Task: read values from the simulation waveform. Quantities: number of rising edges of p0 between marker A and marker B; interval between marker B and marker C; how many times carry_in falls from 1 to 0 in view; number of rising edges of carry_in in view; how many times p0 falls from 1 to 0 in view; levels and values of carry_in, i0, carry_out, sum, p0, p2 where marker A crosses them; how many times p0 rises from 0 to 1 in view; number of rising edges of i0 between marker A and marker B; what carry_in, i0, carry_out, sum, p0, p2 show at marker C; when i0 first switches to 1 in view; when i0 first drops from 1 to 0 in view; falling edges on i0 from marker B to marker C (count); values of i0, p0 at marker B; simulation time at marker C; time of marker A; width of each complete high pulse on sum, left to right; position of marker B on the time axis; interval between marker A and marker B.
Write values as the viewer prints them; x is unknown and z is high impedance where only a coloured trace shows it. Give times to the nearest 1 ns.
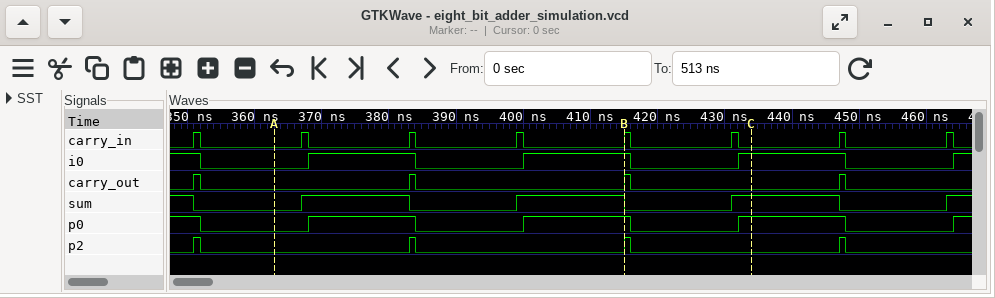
2
19 ns
8
8
4
carry_in=0, i0=0, carry_out=0, sum=0, p0=0, p2=0
4
2
carry_in=0, i0=1, carry_out=0, sum=1, p0=1, p2=0
368 ns
352 ns
1
i0=1, p0=1
434 ns
363 ns
16 ns, 16 ns, 16 ns
415 ns
52 ns
